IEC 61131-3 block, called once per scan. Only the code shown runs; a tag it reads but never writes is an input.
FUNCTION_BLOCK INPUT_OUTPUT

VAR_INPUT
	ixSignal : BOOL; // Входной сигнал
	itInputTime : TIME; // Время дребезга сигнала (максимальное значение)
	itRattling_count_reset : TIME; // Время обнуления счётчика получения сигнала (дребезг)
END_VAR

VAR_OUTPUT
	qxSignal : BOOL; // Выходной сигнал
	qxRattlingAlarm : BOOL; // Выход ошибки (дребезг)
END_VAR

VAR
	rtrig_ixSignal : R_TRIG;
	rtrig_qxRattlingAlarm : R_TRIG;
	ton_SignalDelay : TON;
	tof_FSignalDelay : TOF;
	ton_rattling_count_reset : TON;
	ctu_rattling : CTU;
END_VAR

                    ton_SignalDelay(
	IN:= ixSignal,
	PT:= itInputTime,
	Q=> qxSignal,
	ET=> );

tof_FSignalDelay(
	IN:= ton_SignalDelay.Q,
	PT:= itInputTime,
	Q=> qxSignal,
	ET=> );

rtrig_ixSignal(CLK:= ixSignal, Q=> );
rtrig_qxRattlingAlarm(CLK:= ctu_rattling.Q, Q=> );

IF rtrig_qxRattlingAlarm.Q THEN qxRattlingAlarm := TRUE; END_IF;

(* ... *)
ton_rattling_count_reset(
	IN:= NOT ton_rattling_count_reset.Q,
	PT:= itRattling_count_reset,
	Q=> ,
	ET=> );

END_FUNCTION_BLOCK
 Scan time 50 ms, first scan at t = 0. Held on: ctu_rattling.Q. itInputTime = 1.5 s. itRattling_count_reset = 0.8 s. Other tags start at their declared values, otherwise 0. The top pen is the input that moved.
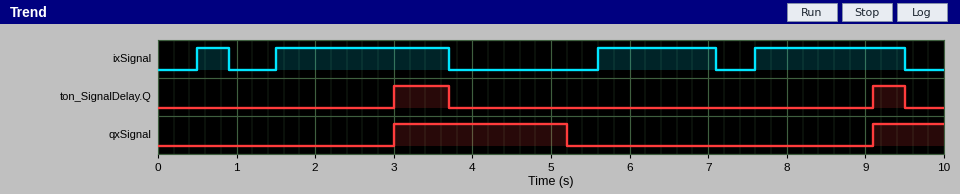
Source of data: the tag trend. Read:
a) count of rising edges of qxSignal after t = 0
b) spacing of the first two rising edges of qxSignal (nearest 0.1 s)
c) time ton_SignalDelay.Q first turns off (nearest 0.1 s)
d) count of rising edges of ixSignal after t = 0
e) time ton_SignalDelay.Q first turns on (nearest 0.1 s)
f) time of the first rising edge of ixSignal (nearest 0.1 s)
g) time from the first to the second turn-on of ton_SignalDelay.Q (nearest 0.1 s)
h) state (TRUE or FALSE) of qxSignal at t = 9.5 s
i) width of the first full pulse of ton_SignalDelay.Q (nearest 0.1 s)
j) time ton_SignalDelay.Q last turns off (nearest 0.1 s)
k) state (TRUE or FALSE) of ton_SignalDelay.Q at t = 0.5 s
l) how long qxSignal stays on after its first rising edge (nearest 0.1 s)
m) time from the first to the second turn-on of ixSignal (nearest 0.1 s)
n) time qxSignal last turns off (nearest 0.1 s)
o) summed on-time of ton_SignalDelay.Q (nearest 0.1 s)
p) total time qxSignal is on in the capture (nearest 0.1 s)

2
6.1 s
3.7 s
4
3.0 s
0.5 s
6.1 s
TRUE
0.7 s
9.5 s
FALSE
2.2 s
1.0 s
5.2 s
1.1 s
3.1 s
